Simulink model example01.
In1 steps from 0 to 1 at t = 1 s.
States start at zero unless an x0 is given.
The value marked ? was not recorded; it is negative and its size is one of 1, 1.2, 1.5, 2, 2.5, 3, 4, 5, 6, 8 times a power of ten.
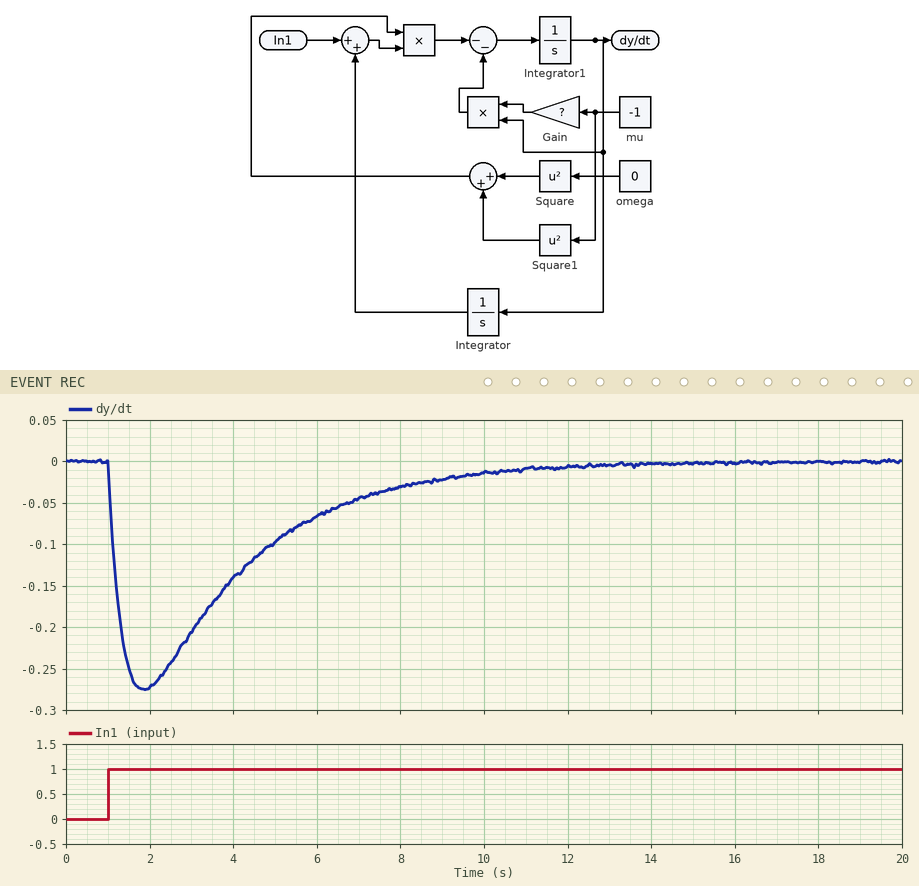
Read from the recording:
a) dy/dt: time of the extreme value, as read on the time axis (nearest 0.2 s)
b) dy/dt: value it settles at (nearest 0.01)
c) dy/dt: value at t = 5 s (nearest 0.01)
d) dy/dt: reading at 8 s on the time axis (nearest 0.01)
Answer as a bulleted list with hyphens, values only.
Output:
- 1.8 s
- 0.00
- -0.10
- -0.03
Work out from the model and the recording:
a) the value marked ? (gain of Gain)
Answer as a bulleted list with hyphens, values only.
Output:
- -3
